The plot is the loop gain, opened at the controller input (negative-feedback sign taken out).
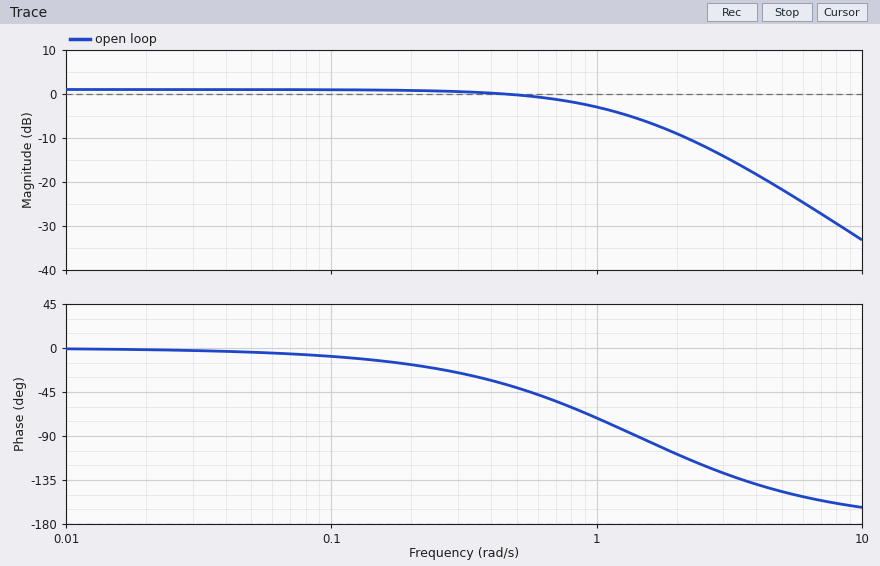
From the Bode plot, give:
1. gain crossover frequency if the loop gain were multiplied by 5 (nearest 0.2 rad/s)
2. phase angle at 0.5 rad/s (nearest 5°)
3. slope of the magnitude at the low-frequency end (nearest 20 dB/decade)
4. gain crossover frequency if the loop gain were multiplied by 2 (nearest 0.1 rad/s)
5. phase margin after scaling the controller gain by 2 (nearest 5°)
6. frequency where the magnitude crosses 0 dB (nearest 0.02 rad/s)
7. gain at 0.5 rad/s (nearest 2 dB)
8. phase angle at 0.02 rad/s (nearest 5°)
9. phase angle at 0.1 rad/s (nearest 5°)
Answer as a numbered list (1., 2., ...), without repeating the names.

1. 3.0 rad/s
2. -40°
3. 0 dB/decade
4. 1.5 rad/s
5. 85°
6. 0.46 rad/s
7. 0 dB
8. 0°
9. -10°
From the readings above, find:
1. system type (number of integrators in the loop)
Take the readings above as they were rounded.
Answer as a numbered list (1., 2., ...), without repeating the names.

1. 0
